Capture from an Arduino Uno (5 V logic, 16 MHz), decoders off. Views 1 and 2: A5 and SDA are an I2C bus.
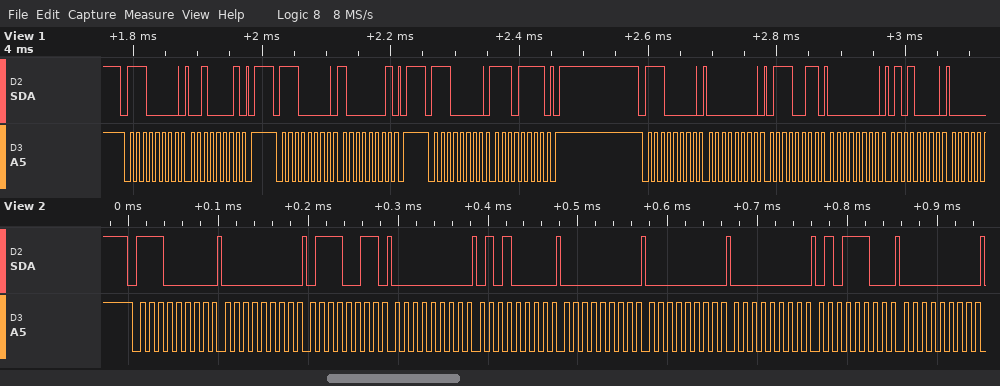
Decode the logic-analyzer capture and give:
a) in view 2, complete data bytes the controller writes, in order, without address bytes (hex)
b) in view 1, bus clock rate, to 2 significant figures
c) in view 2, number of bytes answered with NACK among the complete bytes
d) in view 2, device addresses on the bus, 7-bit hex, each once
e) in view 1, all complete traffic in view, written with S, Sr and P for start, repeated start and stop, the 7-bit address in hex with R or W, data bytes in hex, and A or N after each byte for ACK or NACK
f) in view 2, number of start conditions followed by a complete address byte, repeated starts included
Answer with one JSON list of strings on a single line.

["00 73 00 50 00 00 00 5C 00", "100 kHz", "0", "0x70", "S 70W A 21 A P S 70W A 81 A P S 70W A EF A P S 70W A 00 A 73 A 00 A 50 A", "1"]
